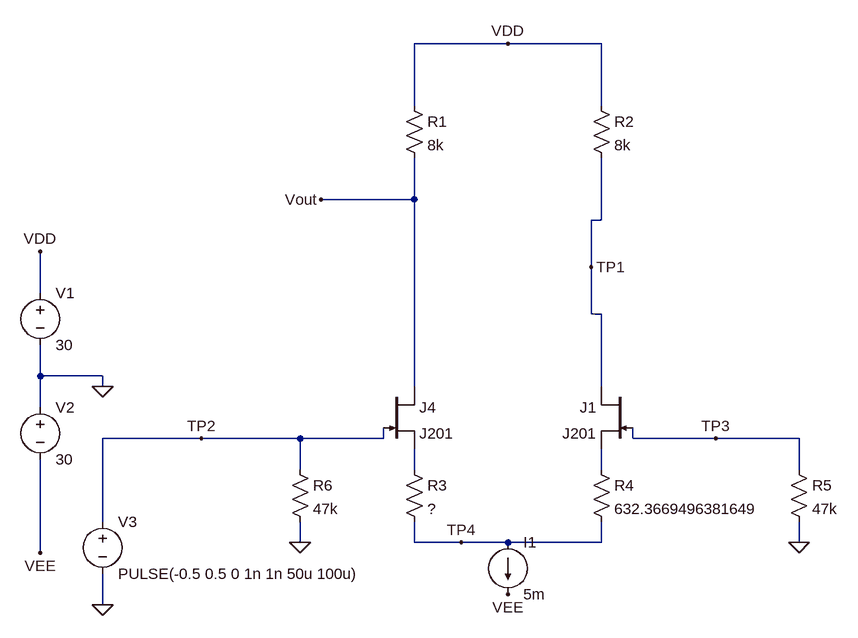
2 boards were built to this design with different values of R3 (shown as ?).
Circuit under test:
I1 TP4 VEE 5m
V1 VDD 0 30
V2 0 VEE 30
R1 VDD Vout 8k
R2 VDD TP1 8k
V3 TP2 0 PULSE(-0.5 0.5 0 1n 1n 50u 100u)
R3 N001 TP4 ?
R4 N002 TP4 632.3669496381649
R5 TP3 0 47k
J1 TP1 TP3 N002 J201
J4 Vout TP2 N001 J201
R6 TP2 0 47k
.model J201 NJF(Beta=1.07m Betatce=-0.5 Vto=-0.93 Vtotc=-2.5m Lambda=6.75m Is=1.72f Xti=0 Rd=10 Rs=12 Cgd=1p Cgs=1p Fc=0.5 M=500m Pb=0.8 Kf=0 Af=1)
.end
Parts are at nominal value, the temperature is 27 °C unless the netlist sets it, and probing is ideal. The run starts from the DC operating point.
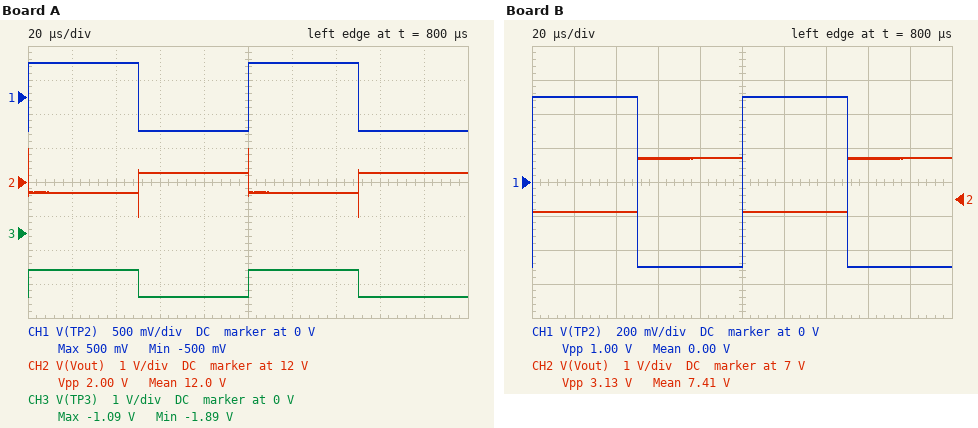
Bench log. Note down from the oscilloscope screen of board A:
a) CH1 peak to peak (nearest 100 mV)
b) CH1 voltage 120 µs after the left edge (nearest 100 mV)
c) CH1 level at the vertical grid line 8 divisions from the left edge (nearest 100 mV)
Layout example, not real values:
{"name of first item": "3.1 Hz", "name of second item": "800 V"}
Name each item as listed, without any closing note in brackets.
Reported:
{"CH1 peak to peak": "1.0 V", "CH1 voltage 120 µs after the left edge": "500 mV", "CH1 level at the vertical grid line 8 divisions from the left edge": "-500 mV"}
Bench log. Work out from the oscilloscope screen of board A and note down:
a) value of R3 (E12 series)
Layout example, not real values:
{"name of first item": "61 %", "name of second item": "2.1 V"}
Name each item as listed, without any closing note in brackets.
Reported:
{"value of R3": "1.5 kΩ"}
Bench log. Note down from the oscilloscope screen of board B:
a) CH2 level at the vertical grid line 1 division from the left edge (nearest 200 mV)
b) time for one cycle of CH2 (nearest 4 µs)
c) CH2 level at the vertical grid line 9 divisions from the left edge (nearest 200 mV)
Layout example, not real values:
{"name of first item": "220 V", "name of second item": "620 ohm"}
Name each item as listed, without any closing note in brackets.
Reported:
{"CH2 level at the vertical grid line 1 division from the left edge": "6.6 V", "time for one cycle of CH2": "100 µs", "CH2 level at the vertical grid line 9 divisions from the left edge": "8.2 V"}
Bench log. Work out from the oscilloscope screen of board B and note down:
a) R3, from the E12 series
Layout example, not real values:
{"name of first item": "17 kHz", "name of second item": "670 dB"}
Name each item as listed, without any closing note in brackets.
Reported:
{"R3, from the E12 series": "270 Ω"}
